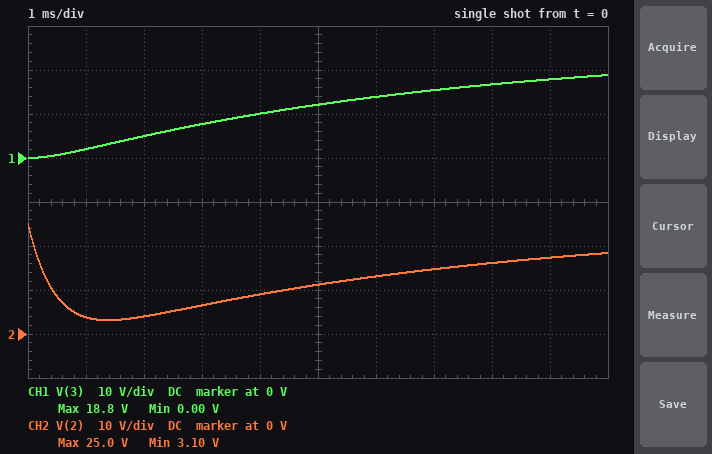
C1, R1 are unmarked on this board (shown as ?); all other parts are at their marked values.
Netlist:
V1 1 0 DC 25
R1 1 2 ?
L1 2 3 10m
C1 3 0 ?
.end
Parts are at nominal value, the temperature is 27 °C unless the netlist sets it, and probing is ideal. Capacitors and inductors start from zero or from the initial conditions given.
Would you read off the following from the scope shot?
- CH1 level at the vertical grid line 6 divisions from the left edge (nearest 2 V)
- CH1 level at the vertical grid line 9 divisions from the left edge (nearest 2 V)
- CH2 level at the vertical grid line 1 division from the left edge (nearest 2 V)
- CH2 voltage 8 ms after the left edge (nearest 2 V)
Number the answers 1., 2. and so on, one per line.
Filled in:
1. 14 V
2. 18 V
3. 4 V
4. 16 V
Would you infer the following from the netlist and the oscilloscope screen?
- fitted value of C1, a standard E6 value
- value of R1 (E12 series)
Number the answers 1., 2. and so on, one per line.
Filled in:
1. 330 µF
2. 22 Ω
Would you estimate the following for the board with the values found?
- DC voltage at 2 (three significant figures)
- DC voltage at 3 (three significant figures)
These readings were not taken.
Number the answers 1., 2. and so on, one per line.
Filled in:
1. 25.0 V
2. 25.0 V
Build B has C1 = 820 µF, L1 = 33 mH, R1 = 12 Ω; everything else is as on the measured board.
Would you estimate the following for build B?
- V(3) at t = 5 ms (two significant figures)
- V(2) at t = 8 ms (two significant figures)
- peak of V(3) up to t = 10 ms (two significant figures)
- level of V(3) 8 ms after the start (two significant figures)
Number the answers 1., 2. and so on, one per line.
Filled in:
1. 6.4 V
2. 8.7 V
3. 15 V
4. 12 V
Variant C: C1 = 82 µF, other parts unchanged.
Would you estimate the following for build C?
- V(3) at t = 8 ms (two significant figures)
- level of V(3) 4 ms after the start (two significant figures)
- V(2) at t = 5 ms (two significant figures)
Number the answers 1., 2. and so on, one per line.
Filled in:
1. 25 V
2. 23 V
3. 24 V
